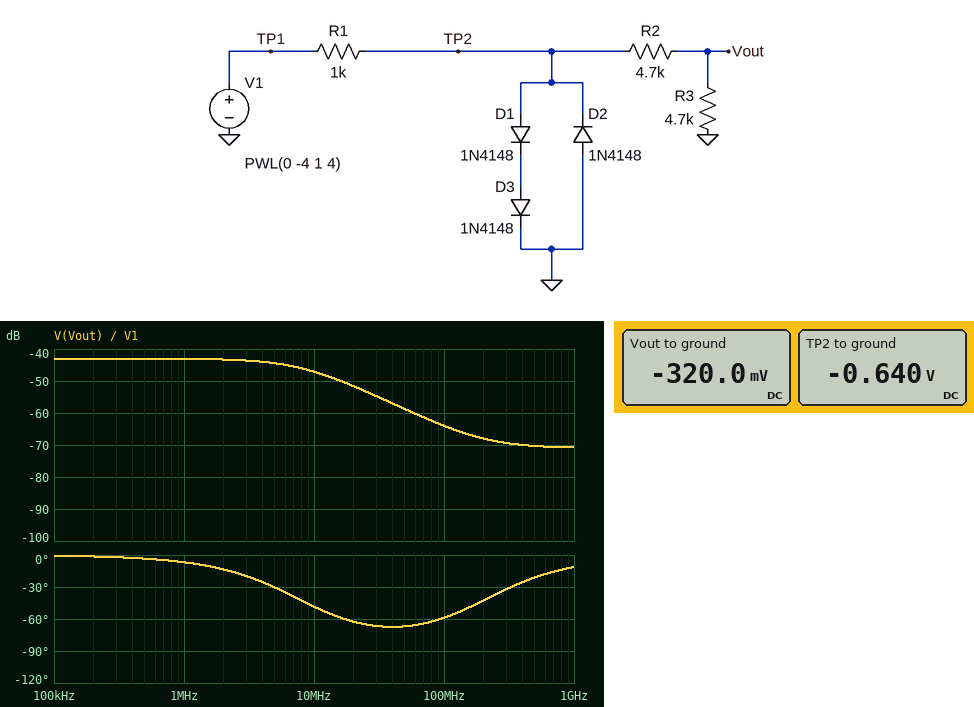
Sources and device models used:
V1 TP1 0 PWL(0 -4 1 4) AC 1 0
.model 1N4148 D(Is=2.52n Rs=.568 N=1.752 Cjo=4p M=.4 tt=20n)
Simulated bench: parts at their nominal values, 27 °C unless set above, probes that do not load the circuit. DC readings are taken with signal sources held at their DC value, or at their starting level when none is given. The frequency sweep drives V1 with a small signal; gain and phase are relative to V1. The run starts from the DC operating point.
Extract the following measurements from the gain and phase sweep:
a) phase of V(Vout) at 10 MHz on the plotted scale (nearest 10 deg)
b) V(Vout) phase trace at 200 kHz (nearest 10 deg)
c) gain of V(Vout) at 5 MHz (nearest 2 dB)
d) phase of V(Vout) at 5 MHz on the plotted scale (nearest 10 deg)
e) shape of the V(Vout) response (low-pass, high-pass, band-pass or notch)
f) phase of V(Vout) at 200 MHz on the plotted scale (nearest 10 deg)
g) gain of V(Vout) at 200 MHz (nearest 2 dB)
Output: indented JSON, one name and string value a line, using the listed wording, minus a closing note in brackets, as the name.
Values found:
{
  "phase of V(Vout) at 10 MHz on the plotted scale": "-50 deg",
  "V(Vout) phase trace at 200 kHz": "0 deg",
  "gain of V(Vout) at 5 MHz": "-44 dB",
  "phase of V(Vout) at 5 MHz on the plotted scale": "-30 deg",
  "shape of the V(Vout) response": "low-pass",
  "phase of V(Vout) at 200 MHz on the plotted scale": "-40 deg",
  "gain of V(Vout) at 200 MHz": "-68 dB"
}
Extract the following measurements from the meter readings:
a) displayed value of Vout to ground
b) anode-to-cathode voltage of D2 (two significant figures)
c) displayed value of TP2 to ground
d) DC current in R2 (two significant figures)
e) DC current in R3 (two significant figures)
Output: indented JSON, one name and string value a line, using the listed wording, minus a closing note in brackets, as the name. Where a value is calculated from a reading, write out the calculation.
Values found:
{
  "displayed value of Vout to ground": "-320.0 mV",
  "anode-to-cathode voltage of D2": "0 V - (-640 mV) = 640 mV",
  "displayed value of TP2 to ground": "-0.640 V",
  "DC current in R2": "(-320 mV - (-640 mV)) / 4.7 kΩ = 68 µA",
  "DC current in R3": "(0 V - (-320 mV)) / 4.7 kΩ = 68 µA"
}
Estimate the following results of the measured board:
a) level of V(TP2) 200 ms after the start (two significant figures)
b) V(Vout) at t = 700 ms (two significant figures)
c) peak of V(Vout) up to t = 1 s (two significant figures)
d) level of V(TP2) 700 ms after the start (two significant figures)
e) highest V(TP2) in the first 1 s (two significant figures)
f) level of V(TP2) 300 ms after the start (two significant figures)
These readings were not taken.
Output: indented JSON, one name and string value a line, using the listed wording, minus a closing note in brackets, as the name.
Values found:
{
  "level of V(TP2) 200 ms after the start": "-610 mV",
  "V(Vout) at t = 700 ms": "540 mV",
  "peak of V(Vout) up to t = 1 s": "630 mV",
  "level of V(TP2) 700 ms after the start": "1.1 V",
  "highest V(TP2) in the first 1 s": "1.3 V",
  "level of V(TP2) 300 ms after the start": "-580 mV"
}
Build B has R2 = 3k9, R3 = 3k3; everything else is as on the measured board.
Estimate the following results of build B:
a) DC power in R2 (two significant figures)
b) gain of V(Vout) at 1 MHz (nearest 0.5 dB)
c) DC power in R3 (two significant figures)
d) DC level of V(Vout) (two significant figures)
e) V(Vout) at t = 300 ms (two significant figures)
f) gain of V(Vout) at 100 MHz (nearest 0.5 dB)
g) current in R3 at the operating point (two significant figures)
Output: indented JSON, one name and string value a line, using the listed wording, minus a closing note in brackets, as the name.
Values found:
{
  "DC power in R2": "31 µW",
  "gain of V(Vout) at 1 MHz": "-44.0 dB",
  "DC power in R3": "26 µW",
  "DC level of V(Vout)": "-290 mV",
  "V(Vout) at t = 300 ms": "-270 mV",
  "gain of V(Vout) at 100 MHz": "-64.5 dB",
  "current in R3 at the operating point": "89 µA"
}
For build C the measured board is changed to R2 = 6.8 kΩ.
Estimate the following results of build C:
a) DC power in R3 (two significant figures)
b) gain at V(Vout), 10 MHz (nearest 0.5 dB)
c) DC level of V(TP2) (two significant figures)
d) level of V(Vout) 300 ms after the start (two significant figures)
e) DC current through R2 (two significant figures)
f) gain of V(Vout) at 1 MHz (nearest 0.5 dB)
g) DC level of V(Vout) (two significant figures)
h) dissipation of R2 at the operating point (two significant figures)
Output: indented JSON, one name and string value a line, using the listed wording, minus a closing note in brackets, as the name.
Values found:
{
  "DC power in R3": "15 µW",
  "gain at V(Vout), 10 MHz": "-49.0 dB",
  "DC level of V(TP2)": "-640 mV",
  "level of V(Vout) 300 ms after the start": "-240 mV",
  "DC current through R2": "56 µA",
  "gain of V(Vout) at 1 MHz": "-45.0 dB",
  "DC level of V(Vout)": "-260 mV",
  "dissipation of R2 at the operating point": "21 µW"
}
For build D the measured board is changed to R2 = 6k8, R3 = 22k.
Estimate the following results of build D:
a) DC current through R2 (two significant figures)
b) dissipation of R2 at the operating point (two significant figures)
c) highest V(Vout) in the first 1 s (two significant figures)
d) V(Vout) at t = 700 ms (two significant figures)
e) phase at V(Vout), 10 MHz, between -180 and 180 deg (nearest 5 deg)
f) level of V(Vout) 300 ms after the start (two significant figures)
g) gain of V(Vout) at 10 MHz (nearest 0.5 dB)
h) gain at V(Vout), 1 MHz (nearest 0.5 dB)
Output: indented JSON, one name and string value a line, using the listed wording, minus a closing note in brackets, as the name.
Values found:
{
  "DC current through R2": "22 µA",
  "dissipation of R2 at the operating point": "3.4 µW",
  "highest V(Vout) in the first 1 s": "960 mV",
  "V(Vout) at t = 700 ms": "840 mV",
  "phase at V(Vout), 10 MHz, between -180 and 180 deg": "-50 deg",
  "level of V(Vout) 300 ms after the start": "-450 mV",
  "gain of V(Vout) at 10 MHz": "-43.5 dB",
  "gain at V(Vout), 1 MHz": "-39.5 dB"
}
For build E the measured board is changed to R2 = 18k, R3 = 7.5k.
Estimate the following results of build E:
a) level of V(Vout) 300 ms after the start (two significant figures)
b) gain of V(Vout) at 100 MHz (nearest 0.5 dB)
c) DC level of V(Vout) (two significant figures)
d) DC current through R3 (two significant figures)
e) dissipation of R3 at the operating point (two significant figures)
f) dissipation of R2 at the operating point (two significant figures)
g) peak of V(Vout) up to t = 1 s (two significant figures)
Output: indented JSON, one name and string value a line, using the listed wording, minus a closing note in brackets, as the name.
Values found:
{
  "level of V(Vout) 300 ms after the start": "-170 mV",
  "gain of V(Vout) at 100 MHz": "-68.5 dB",
  "DC level of V(Vout)": "-190 mV",
  "DC current through R3": "25 µA",
  "dissipation of R3 at the operating point": "4.7 µW",
  "dissipation of R2 at the operating point": "11 µW",
  "peak of V(Vout) up to t = 1 s": "370 mV"
}
